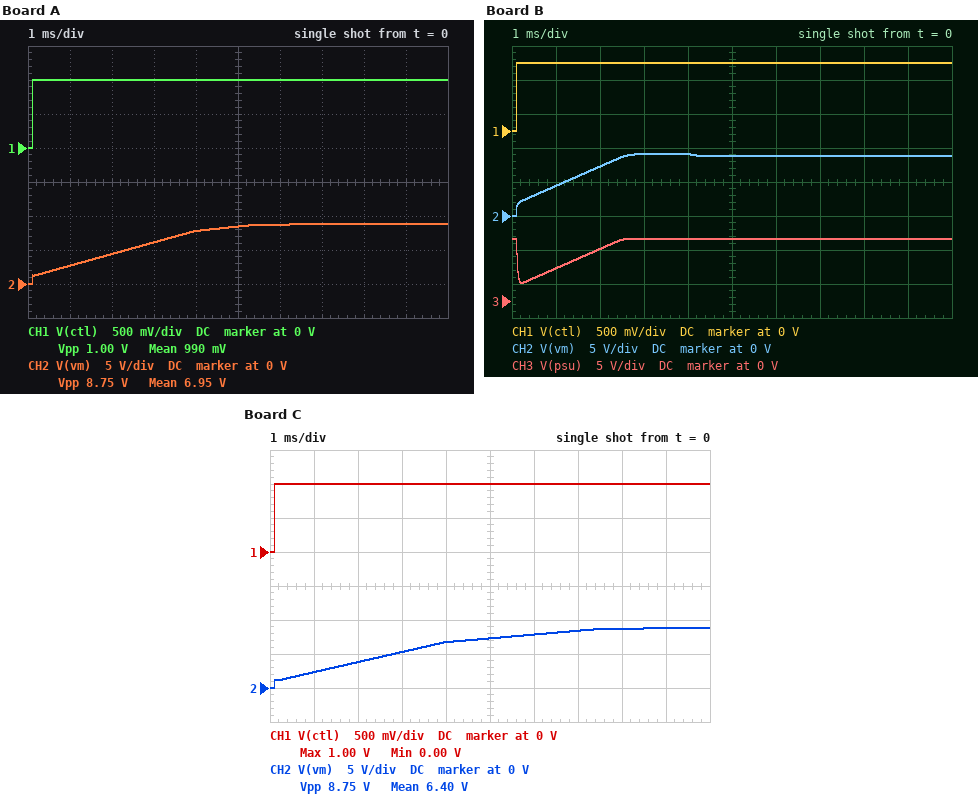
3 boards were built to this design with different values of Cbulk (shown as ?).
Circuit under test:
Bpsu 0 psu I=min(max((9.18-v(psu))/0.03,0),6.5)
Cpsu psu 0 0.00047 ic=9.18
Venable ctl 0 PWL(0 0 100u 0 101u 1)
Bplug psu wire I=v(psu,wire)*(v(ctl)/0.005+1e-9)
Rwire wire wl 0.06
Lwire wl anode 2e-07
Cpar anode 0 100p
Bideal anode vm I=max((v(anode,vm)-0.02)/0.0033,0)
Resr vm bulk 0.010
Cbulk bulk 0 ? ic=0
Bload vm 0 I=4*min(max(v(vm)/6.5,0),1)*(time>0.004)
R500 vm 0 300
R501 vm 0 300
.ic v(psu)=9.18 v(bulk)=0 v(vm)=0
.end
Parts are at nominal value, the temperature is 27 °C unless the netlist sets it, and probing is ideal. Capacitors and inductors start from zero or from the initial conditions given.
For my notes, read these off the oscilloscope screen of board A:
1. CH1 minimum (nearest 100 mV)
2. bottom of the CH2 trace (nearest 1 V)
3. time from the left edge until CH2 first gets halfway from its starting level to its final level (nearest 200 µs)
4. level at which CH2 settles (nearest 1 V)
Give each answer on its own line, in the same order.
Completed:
0 V
0 V
2.0 ms
9 V
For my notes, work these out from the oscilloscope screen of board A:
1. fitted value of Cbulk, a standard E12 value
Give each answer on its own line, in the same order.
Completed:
3.3 mF
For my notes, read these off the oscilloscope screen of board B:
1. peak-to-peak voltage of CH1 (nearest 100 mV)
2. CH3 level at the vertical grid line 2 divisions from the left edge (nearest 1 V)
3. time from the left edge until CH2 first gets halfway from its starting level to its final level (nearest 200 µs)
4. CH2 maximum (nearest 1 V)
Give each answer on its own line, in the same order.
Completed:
1.0 V
8 V
1.0 ms
9 V
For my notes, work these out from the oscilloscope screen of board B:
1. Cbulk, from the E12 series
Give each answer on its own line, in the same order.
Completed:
1.8 mF
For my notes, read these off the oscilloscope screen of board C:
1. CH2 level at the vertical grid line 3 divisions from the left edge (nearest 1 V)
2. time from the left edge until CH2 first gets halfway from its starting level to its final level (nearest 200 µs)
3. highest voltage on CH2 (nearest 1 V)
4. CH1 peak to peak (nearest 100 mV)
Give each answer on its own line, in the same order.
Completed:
5 V
2.4 ms
9 V
1.0 V
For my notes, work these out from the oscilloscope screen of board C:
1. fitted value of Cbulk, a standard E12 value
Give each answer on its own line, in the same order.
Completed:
3.9 mF
